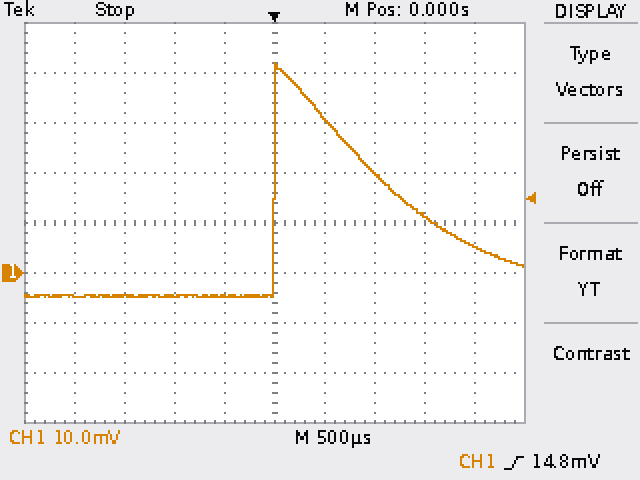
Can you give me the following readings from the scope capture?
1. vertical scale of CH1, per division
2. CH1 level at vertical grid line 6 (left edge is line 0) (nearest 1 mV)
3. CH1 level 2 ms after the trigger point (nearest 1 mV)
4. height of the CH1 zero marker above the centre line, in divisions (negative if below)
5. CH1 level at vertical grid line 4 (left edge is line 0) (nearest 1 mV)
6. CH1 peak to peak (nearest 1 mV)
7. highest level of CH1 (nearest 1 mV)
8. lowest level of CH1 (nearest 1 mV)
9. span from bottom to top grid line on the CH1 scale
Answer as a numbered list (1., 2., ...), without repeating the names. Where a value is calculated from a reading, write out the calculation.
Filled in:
1. 10 mV
2. 31 mV
3. 5 mV
4. -1.0 div
5. -5 mV
6. 42 mV − (-5 mV) = 47 mV
7. 42 mV
8. -5 mV
9. 80 mV
